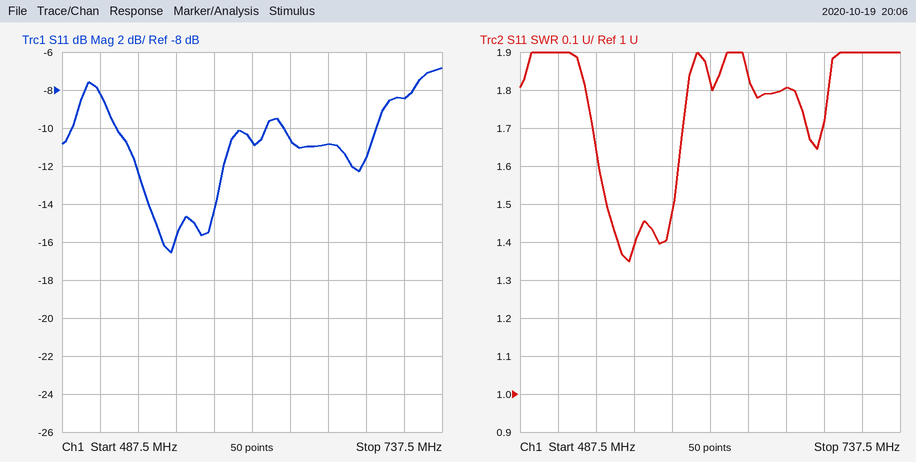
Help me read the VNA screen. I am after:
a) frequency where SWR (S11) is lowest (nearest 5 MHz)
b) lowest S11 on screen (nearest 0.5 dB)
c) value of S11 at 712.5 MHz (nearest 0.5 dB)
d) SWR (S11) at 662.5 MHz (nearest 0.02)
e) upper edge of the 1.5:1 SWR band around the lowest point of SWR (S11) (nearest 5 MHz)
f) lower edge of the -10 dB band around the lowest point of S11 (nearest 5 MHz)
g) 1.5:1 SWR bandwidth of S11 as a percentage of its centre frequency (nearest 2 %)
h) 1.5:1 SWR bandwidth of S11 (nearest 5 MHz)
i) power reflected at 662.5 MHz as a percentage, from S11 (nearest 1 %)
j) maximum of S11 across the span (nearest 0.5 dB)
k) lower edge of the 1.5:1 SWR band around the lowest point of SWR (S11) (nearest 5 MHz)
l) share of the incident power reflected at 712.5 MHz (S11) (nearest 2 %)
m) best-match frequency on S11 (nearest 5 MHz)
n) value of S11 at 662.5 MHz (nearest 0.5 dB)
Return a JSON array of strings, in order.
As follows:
["560 MHz", "-16.5 dB", "-8.5 dB", "1.80", "590 MHz", "525 MHz", "8 %", "45 MHz", "8 %", "-7.0 dB", "545 MHz", "14 %", "560 MHz", "-11.0 dB"]
